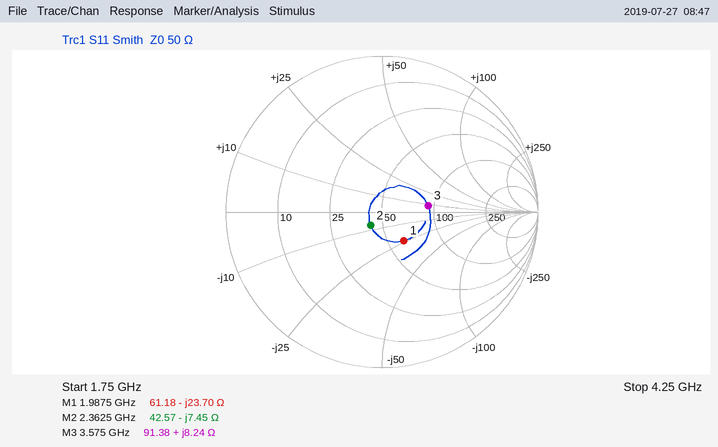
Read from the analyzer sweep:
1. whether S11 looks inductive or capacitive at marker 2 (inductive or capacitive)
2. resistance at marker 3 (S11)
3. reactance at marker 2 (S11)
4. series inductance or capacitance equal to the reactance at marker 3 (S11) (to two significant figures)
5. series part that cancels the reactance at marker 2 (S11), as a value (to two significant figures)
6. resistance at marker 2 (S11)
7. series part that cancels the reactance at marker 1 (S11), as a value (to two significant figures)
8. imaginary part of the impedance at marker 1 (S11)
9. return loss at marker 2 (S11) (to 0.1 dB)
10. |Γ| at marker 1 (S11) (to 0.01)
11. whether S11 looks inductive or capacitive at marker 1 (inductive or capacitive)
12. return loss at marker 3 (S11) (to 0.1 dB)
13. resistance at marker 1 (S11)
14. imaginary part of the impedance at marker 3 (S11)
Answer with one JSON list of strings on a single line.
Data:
["capacitive", "91.38 Ω", "-7.45 Ω", "370 pH", "500 pH", "42.57 Ω", "1.9 nH", "-23.70 Ω", "18.9 dB", "0.23", "capacitive", "10.5 dB", "61.18 Ω", "+8.24 Ω"]
